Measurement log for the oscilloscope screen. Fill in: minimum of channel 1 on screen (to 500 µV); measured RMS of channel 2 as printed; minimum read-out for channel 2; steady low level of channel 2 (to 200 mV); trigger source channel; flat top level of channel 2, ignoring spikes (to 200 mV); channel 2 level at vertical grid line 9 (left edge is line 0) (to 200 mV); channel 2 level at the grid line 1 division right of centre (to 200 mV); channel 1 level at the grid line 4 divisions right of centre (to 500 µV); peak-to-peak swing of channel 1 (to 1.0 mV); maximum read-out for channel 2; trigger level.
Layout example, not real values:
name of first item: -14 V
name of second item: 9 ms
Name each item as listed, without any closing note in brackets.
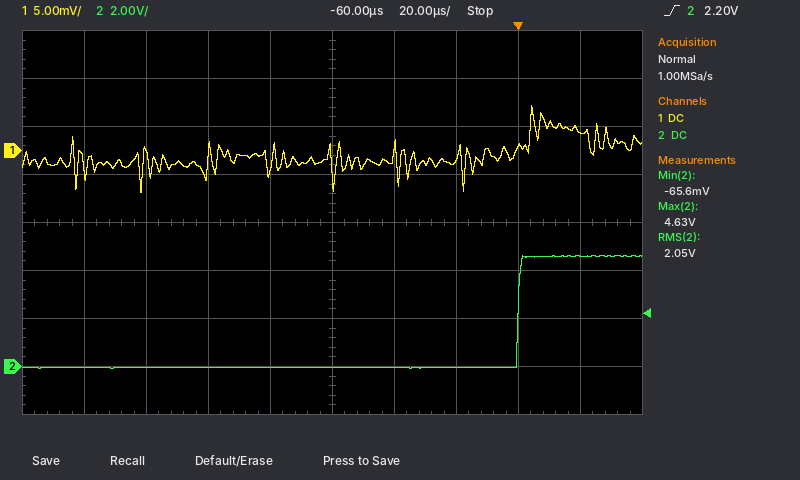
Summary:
minimum of channel 1 on screen: -4.5 mV
measured RMS of channel 2 as printed: 2.05 V
minimum read-out for channel 2: -65.6 mV
steady low level of channel 2: 0.0 V
trigger source channel: channel 2
flat top level of channel 2, ignoring spikes: 4.6 V
channel 2 level at vertical grid line 9 (left edge is line 0): 4.6 V
channel 2 level at the grid line 1 division right of centre: 0.0 V
channel 1 level at the grid line 4 divisions right of centre: 2.0 mV
peak-to-peak swing of channel 1: 9.0 mV
maximum read-out for channel 2: 4.63 V
trigger level: 2.20 V
